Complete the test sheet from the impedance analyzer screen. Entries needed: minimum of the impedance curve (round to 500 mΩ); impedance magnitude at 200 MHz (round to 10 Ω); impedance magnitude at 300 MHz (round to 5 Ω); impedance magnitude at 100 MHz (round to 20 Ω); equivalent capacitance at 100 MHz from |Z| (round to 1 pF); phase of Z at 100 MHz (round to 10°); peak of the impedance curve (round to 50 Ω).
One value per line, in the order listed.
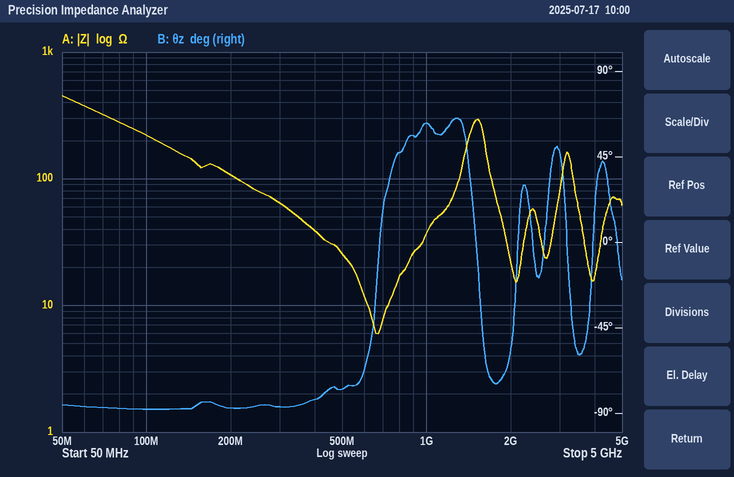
6.0 Ω
110 Ω
65 Ω
220 Ω
7 pF
-90°
450 Ω
